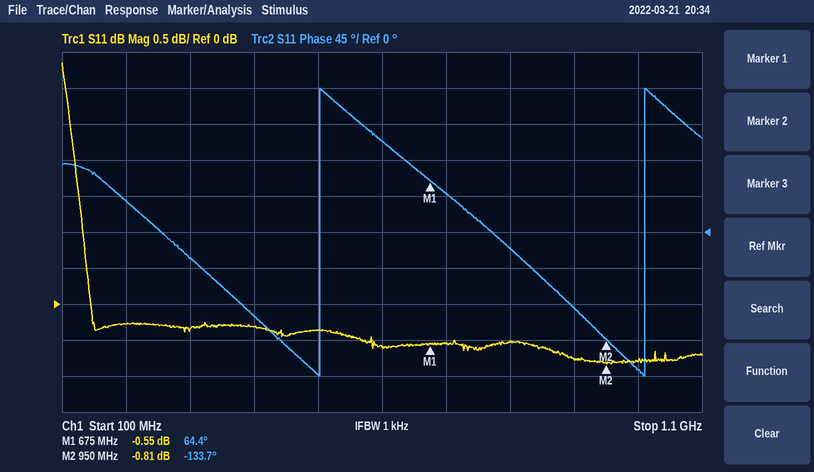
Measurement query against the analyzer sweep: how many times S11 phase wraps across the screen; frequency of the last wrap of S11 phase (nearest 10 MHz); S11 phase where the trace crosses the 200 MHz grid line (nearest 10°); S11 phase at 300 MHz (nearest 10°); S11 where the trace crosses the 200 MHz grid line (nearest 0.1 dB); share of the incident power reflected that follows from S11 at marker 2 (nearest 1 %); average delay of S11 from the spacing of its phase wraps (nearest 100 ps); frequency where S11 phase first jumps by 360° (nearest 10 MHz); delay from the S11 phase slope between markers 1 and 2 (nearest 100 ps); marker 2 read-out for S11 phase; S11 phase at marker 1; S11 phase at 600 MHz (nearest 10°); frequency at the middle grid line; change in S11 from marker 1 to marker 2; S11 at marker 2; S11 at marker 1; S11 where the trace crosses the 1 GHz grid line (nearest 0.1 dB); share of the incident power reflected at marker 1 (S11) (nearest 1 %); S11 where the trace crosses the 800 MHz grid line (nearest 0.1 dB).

2
1.01 GHz
40°
-30°
-0.3 dB
83 %
2.0 ns
500 MHz
2.0 ns
-133.7°
64.4°
110°
600 MHz
-0.26 dB
-0.81 dB
-0.55 dB
-0.8 dB
88 %
-0.5 dB
